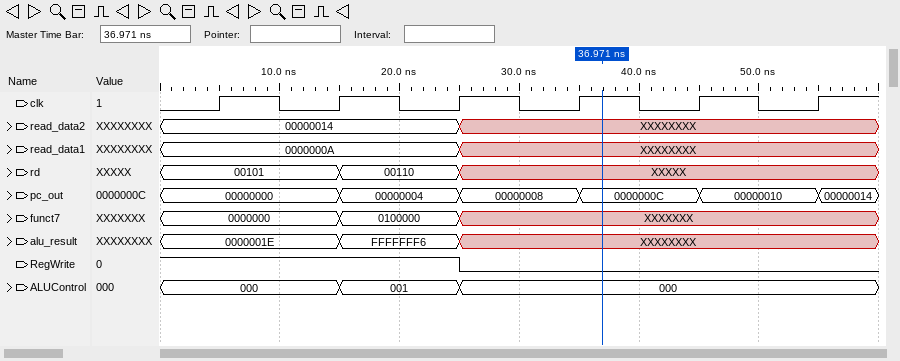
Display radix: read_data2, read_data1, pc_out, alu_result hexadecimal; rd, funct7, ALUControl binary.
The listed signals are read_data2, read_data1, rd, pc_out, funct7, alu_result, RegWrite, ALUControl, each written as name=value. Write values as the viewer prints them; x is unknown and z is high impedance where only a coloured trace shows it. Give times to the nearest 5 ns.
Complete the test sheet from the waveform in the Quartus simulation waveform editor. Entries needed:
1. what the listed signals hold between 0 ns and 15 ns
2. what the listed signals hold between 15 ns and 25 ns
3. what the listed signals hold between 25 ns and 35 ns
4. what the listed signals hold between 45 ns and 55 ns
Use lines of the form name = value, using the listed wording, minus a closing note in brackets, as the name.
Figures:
what the listed signals hold between 0 ns and 15 ns = read_data2=00000014, read_data1=0000000A, rd=00101, pc_out=00000000, funct7=0000000, alu_result=0000001E, RegWrite=1, ALUControl=000
what the listed signals hold between 15 ns and 25 ns = read_data2=00000014, read_data1=0000000A, rd=00110, pc_out=00000004, funct7=0100000, alu_result=FFFFFFF6, RegWrite=1, ALUControl=001
what the listed signals hold between 25 ns and 35 ns = read_data2=XXXXXXXX, read_data1=XXXXXXXX, rd=XXXXX, pc_out=00000008, funct7=XXXXXXX, alu_result=XXXXXXXX, RegWrite=0, ALUControl=000
what the listed signals hold between 45 ns and 55 ns = read_data2=XXXXXXXX, read_data1=XXXXXXXX, rd=XXXXX, pc_out=00000010, funct7=XXXXXXX, alu_result=XXXXXXXX, RegWrite=0, ALUControl=000
